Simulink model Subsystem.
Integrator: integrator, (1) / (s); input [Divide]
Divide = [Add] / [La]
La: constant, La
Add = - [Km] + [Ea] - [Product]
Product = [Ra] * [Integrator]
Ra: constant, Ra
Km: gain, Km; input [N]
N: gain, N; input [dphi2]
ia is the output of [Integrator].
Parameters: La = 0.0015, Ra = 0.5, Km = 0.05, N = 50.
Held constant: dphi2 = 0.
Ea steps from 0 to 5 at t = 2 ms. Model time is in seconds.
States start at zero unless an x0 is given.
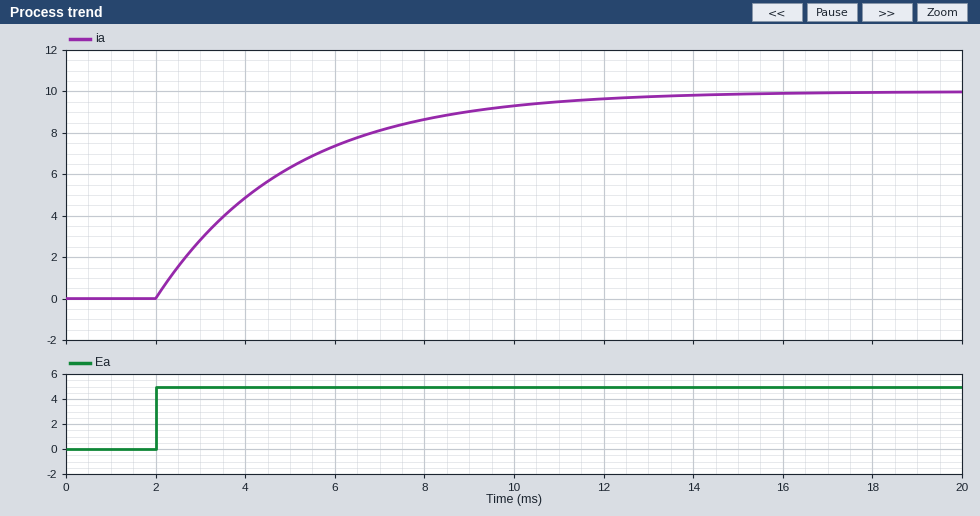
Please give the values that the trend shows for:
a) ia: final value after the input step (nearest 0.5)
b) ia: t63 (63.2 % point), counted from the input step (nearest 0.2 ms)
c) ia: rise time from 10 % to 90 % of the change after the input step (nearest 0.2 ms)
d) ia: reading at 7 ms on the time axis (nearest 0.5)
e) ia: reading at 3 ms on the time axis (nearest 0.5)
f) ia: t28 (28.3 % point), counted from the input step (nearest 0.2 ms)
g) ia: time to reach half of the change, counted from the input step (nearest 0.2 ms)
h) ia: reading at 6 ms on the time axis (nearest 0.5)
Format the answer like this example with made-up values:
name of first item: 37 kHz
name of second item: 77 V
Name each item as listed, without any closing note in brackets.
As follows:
ia: final value after the input step: 10.0
ia: t63 (63.2 % point), counted from the input step: 3.0 ms
ia: rise time from 10 % to 90 % of the change after the input step: 6.6 ms
ia: reading at 7 ms on the time axis: 8.0
ia: reading at 3 ms on the time axis: 3.0
ia: t28 (28.3 % point), counted from the input step: 1.0 ms
ia: time to reach half of the change, counted from the input step: 2.0 ms
ia: reading at 6 ms on the time axis: 7.5
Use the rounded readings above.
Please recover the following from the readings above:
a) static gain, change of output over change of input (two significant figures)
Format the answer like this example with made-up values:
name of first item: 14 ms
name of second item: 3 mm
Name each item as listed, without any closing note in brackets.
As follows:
static gain, change of output over change of input: 2.0
